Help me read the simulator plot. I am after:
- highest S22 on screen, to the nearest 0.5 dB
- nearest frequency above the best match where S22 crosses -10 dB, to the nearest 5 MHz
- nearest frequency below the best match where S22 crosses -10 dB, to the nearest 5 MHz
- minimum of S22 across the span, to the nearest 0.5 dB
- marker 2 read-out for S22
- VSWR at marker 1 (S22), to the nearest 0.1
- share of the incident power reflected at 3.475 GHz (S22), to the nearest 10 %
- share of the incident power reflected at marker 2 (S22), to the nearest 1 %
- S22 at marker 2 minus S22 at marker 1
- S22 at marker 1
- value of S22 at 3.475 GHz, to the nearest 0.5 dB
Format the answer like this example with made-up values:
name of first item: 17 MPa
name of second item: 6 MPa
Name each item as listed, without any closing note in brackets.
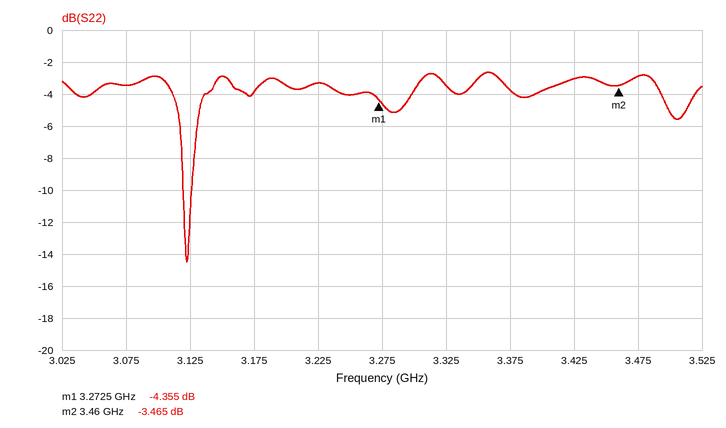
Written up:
highest S22 on screen, to the nearest 0.5 dB: -2.5 dB
nearest frequency above the best match where S22 crosses -10 dB, to the nearest 5 MHz: 3.125 GHz
nearest frequency below the best match where S22 crosses -10 dB, to the nearest 5 MHz: 3.120 GHz
minimum of S22 across the span, to the nearest 0.5 dB: -14.5 dB
marker 2 read-out for S22: -3.465 dB
VSWR at marker 1 (S22), to the nearest 0.1: 4.1
share of the incident power reflected at 3.475 GHz (S22), to the nearest 10 %: 50 %
share of the incident power reflected at marker 2 (S22), to the nearest 1 %: 45 %
S22 at marker 2 minus S22 at marker 1: 0.890 dB
S22 at marker 1: -4.355 dB
value of S22 at 3.475 GHz, to the nearest 0.5 dB: -3.0 dB
